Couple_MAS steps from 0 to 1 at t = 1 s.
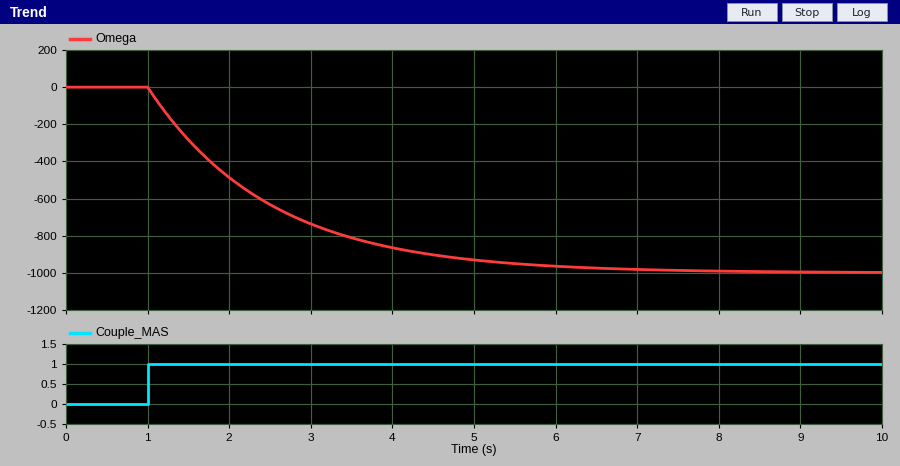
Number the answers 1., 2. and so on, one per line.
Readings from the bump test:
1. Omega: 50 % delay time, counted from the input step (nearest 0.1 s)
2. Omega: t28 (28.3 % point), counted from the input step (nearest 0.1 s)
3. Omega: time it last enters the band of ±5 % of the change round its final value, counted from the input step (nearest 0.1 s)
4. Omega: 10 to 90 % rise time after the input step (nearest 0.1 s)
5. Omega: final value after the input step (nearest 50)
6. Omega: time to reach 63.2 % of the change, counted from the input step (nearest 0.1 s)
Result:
1. 1.0 s
2. 0.5 s
3. 4.5 s
4. 3.3 s
5. -1000
6. 1.5 s
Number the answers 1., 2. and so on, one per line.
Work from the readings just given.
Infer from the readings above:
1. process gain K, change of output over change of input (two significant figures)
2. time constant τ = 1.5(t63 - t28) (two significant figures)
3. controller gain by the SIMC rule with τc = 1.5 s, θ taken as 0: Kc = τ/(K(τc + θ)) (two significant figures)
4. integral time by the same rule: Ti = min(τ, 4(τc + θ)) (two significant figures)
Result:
1. -1000
2. 1.5 s
3. -0.0010
4. 1.5 s
